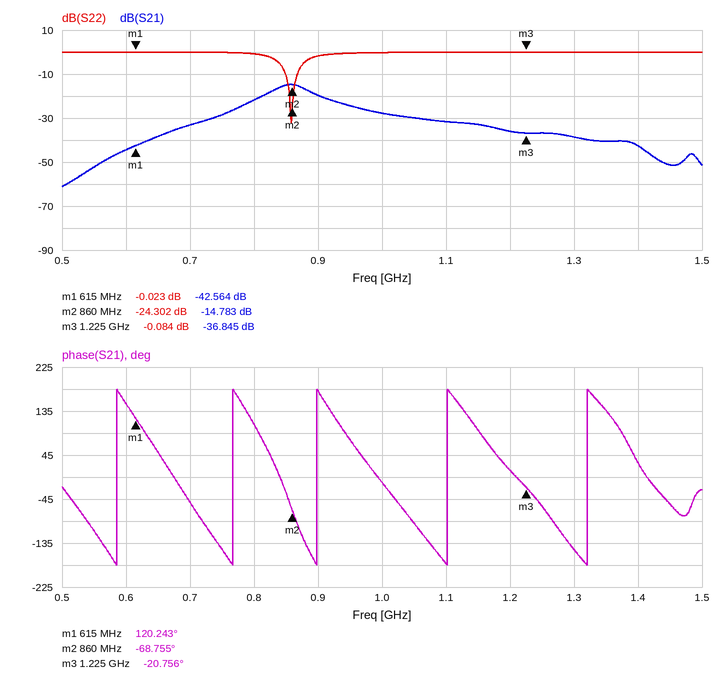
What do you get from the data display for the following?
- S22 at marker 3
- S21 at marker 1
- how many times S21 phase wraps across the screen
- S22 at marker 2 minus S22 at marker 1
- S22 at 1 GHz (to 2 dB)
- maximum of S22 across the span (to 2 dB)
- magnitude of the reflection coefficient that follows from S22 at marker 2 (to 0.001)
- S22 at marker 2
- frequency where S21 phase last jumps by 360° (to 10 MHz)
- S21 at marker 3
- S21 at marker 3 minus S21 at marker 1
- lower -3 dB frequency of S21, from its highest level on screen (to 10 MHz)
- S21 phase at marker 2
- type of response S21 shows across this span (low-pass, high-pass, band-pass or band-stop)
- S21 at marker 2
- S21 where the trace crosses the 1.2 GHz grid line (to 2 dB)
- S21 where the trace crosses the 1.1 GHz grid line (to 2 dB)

-0.084 dB
-42.564 dB
5
-24.279 dB
0 dB
0 dB
0.061
-24.302 dB
1.32 GHz
-36.845 dB
5.719 dB
830 MHz
-68.755°
band-pass
-14.783 dB
-36 dB
-32 dB
